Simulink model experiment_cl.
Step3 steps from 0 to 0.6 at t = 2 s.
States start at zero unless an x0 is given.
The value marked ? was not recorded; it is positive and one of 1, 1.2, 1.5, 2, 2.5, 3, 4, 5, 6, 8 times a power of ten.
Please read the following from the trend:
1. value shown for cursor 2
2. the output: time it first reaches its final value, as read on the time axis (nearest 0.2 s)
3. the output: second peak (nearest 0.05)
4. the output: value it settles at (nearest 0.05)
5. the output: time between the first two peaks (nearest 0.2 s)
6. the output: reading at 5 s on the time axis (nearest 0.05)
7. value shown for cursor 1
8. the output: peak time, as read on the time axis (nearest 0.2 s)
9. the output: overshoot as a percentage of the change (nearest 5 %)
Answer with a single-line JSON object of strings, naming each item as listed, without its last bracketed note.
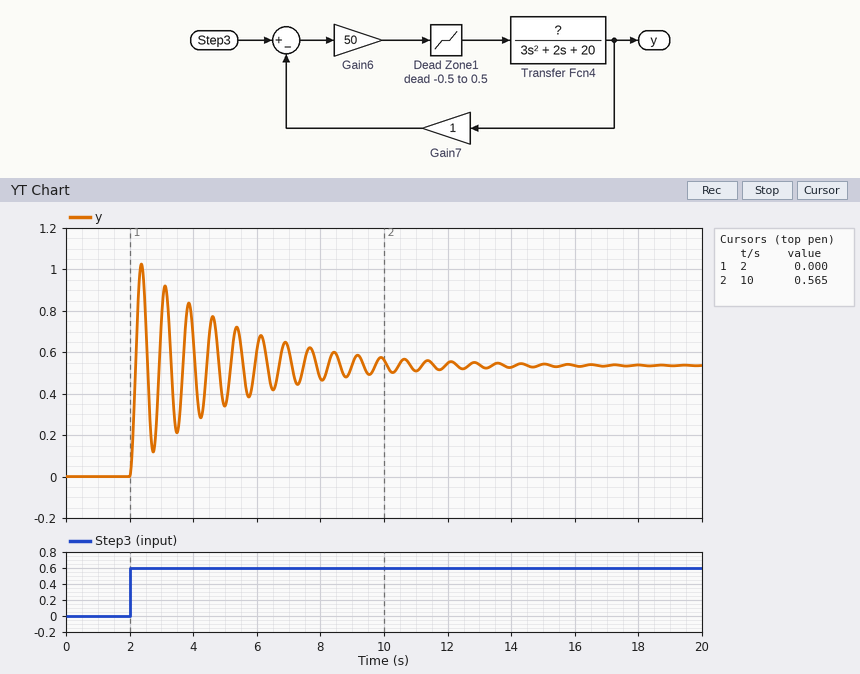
{"value shown for cursor 2": "0.565", "the output: time it first reaches its final value, as read on the time axis": "2.2 s", "the output: second peak": "0.90", "the output: value it settles at": "0.55", "the output: time between the first two peaks": "0.8 s", "the output: reading at 5 s on the time axis": "0.35", "value shown for cursor 1": "0.000", "the output: peak time, as read on the time axis": "2.4 s", "the output: overshoot as a percentage of the change": "90 %"}
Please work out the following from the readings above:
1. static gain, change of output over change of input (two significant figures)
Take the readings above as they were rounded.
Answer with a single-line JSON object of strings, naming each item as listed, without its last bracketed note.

{"static gain, change of output over change of input": "0.92"}
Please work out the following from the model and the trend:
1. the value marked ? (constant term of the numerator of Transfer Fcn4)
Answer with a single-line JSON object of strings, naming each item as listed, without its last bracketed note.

{"the value marked ?": "4"}
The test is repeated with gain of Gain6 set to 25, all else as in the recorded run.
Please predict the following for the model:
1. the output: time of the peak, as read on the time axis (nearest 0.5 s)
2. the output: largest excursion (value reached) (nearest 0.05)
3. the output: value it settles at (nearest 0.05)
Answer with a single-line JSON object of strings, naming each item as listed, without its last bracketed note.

{"the output: time of the peak, as read on the time axis": "2.5 s", "the output: largest excursion (value reached)": "0.90", "the output: value it settles at": "0.50"}
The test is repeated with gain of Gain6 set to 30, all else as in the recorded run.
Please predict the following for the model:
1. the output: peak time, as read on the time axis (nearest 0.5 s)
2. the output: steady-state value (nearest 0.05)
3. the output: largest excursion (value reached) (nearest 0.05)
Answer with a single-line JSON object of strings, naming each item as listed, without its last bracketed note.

{"the output: peak time, as read on the time axis": "2.5 s", "the output: steady-state value": "0.50", "the output: largest excursion (value reached)": "0.95"}
